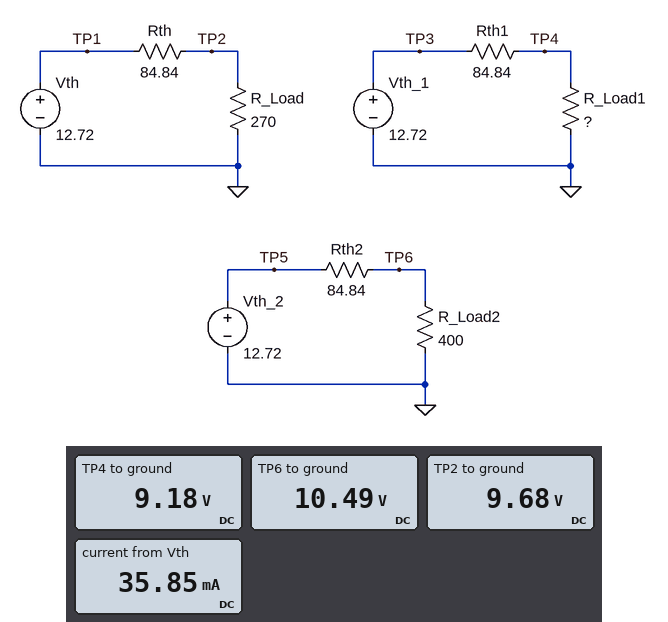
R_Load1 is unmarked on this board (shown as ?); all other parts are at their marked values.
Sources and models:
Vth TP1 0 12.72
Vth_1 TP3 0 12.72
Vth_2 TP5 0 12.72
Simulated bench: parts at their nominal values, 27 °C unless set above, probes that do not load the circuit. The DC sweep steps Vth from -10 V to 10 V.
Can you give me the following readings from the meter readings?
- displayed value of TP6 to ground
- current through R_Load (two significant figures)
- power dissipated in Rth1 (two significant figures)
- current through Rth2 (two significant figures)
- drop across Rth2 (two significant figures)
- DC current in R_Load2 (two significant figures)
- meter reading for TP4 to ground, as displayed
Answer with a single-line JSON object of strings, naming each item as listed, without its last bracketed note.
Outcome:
{"displayed value of TP6 to ground": "10.49 V", "current through R_Load": "36 mA", "power dissipated in Rth1": "150 mW", "current through Rth2": "26 mA", "drop across Rth2": "2.2 V", "DC current in R_Load2": "26 mA", "meter reading for TP4 to ground, as displayed": "9.18 V"}
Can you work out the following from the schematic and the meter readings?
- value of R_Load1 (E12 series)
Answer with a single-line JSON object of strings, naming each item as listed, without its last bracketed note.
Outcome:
{"value of R_Load1": "220 Ω"}
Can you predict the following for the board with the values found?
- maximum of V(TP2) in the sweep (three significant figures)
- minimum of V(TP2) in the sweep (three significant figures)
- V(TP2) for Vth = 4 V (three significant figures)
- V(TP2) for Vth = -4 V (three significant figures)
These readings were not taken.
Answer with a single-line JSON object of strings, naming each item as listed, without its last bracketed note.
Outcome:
{"maximum of V(TP2) in the sweep": "7.61 V", "minimum of V(TP2) in the sweep": "-7.61 V", "V(TP2) for Vth = 4 V": "3.04 V", "V(TP2) for Vth = -4 V": "-3.04 V"}
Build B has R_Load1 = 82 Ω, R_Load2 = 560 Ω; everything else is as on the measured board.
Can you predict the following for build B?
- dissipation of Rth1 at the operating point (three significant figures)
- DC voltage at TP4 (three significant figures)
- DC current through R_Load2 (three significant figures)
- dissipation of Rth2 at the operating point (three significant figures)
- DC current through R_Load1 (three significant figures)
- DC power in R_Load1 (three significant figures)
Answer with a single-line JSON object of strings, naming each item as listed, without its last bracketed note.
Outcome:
{"dissipation of Rth1 at the operating point": "493 mW", "DC voltage at TP4": "6.25 V", "DC current through R_Load2": "19.7 mA", "dissipation of Rth2 at the operating point": "33.0 mW", "DC current through R_Load1": "76.2 mA", "DC power in R_Load1": "477 mW"}
